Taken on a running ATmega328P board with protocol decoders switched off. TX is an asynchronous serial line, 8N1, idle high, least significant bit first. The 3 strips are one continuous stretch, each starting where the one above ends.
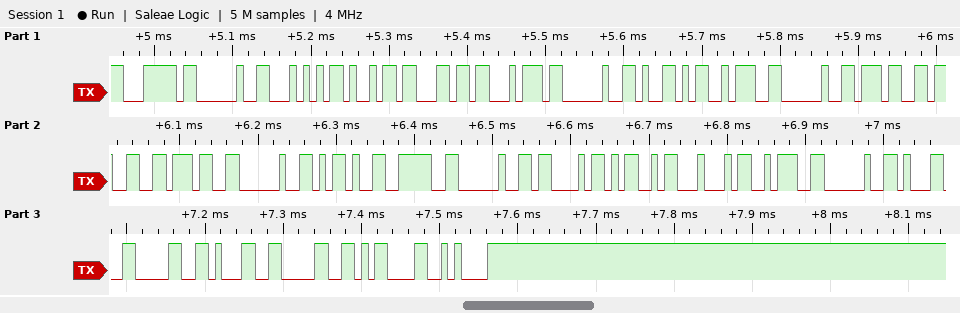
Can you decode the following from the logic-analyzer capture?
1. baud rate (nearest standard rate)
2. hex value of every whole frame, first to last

115200 baud
0x7C 0x20 0x54 0x69 0x6C 0x74 0x20 0x59 0x3A 0x20 0x37 0x33 0x37 0x20 0x2D 0x3E 0x20 0x43 0x4D 0x44 0x3A 0x20 0x31 0x30 0x31 0x30 0x0D 0x0A
